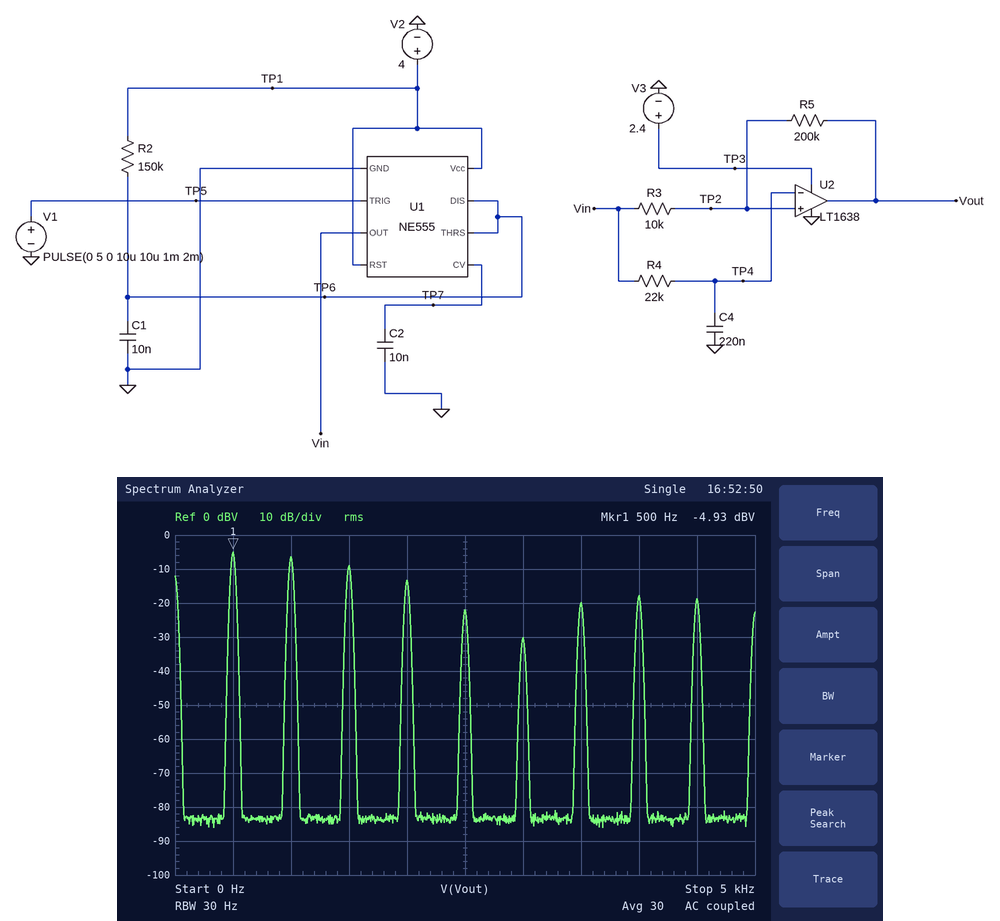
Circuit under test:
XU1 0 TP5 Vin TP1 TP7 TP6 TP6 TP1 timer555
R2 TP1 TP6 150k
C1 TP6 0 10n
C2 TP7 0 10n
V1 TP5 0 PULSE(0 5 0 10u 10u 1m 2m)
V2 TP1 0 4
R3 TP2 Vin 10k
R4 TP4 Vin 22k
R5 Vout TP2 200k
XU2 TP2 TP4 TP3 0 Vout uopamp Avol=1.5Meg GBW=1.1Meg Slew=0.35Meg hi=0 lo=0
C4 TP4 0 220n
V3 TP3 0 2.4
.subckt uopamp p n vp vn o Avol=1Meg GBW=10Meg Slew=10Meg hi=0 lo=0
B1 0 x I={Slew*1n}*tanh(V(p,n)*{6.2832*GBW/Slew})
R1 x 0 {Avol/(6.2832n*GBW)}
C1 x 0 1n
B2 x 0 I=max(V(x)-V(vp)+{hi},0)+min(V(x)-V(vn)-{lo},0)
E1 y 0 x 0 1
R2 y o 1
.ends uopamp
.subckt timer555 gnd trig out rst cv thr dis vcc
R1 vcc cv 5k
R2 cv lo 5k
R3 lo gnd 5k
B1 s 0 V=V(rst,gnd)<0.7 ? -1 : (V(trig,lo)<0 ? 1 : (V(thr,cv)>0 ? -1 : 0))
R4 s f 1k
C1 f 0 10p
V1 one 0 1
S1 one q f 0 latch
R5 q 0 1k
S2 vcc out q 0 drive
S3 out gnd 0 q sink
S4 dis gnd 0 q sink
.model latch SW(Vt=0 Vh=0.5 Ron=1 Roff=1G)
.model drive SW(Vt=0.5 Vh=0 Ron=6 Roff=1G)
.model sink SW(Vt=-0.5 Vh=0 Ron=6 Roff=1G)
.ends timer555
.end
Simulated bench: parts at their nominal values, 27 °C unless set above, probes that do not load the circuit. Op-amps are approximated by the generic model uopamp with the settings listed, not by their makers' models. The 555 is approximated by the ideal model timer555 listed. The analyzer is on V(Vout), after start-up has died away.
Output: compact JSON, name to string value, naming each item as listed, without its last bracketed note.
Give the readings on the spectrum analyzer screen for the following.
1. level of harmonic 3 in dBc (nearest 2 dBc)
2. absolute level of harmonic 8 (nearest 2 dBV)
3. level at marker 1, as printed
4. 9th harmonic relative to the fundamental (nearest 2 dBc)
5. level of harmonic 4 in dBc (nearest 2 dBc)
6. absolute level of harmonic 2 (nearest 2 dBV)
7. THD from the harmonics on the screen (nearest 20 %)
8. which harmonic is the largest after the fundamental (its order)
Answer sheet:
{"level of harmonic 3 in dBc": "-4 dBc", "absolute level of harmonic 8": "-18 dBV", "level at marker 1, as printed": "-4.93 dBV", "9th harmonic relative to the fundamental": "-14 dBc", "level of harmonic 4 in dBc": "-8 dBc", "absolute level of harmonic 2": "-6 dBV", "THD from the harmonics on the screen": "120 %", "which harmonic is the largest after the fundamental": "2"}
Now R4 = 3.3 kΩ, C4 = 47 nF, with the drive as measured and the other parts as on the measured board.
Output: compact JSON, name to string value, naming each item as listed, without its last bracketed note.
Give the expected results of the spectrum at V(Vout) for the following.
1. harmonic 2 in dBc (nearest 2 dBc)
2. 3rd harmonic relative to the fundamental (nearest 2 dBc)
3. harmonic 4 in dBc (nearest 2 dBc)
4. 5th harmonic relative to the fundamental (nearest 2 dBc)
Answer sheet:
{"harmonic 2 in dBc": "-4 dBc", "3rd harmonic relative to the fundamental": "-18 dBc", "harmonic 4 in dBc": "-14 dBc", "5th harmonic relative to the fundamental": "-12 dBc"}
